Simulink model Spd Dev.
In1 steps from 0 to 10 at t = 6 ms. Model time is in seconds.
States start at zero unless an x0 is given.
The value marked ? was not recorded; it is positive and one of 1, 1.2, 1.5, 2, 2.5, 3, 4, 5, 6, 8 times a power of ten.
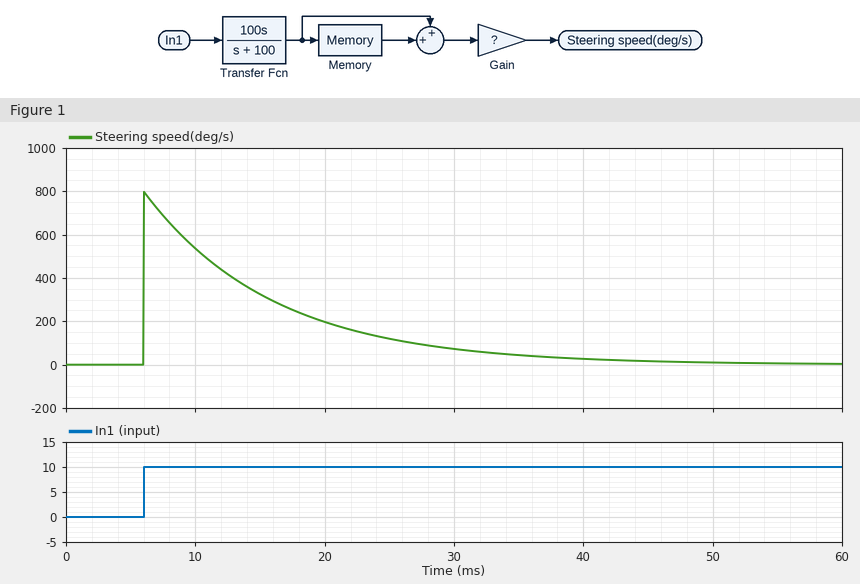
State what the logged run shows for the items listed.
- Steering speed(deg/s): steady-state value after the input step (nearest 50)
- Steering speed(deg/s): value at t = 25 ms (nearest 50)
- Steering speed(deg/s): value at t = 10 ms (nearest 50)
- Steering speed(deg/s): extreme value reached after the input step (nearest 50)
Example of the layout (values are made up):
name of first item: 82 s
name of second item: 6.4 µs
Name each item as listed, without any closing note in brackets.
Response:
Steering speed(deg/s): steady-state value after the input step: 0
Steering speed(deg/s): value at t = 25 ms: 100
Steering speed(deg/s): value at t = 10 ms: 550
Steering speed(deg/s): extreme value reached after the input step: 800
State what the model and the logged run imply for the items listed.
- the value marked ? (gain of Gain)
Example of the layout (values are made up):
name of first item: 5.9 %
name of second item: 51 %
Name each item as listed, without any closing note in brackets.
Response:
the value marked ?: 0.4
